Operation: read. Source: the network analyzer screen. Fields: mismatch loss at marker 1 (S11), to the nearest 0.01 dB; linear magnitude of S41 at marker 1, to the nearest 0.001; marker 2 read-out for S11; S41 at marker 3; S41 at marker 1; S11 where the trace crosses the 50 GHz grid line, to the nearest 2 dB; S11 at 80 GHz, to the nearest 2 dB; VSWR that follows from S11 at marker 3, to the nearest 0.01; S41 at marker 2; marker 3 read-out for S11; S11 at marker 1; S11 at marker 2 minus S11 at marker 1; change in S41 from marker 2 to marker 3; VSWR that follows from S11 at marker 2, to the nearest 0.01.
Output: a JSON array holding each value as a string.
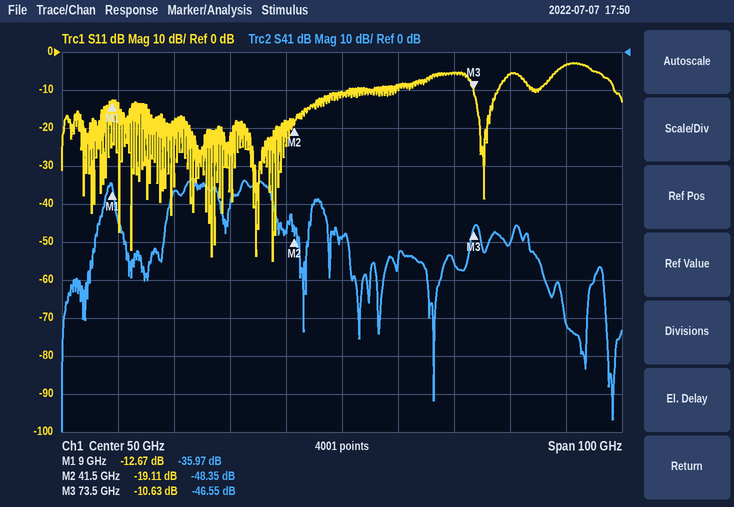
["0.24 dB", "0.016", "-19.11 dB", "-46.55 dB", "-35.97 dB", "-10 dB", "-6 dB", "1.83", "-48.35 dB", "-10.63 dB", "-12.67 dB", "-6.44 dB", "1.80 dB", "1.25"]
